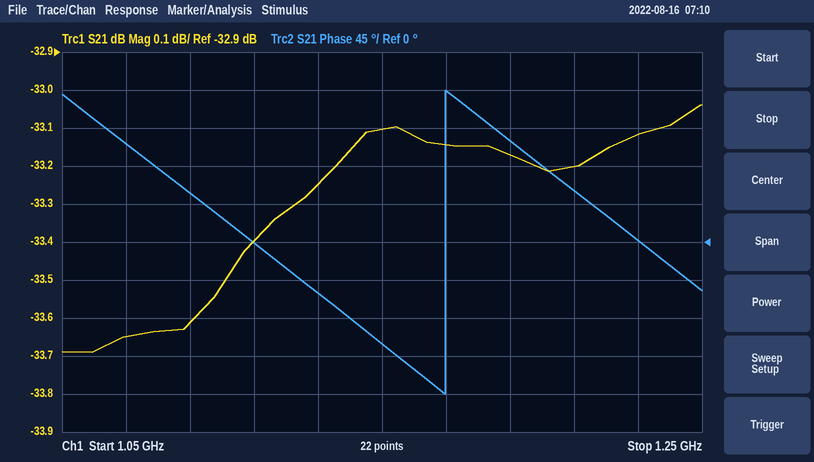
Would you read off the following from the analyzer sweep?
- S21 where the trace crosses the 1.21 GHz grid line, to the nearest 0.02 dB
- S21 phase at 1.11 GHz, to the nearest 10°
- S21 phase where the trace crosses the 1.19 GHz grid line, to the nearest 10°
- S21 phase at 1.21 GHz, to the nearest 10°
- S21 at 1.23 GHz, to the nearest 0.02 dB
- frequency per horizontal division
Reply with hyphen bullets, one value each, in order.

- -33.20 dB
- 0°
- 120°
- 60°
- -33.12 dB
- 20 MHz
